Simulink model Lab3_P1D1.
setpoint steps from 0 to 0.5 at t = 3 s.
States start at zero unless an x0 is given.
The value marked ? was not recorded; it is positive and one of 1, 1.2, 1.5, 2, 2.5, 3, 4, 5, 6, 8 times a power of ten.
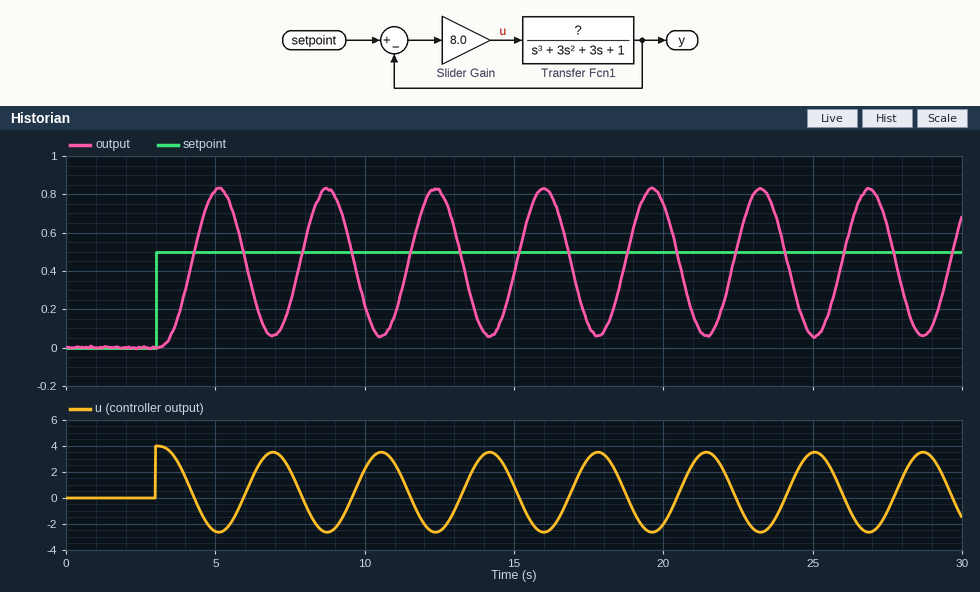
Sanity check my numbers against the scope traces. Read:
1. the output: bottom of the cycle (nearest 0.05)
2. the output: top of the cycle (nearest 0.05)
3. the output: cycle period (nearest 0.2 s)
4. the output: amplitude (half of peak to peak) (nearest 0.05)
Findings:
0.05
0.85
3.6 s
0.40
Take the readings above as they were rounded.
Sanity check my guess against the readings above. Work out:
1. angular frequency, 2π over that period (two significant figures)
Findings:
1.7 rad/s
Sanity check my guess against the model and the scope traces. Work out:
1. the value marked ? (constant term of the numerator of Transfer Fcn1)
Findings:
1
